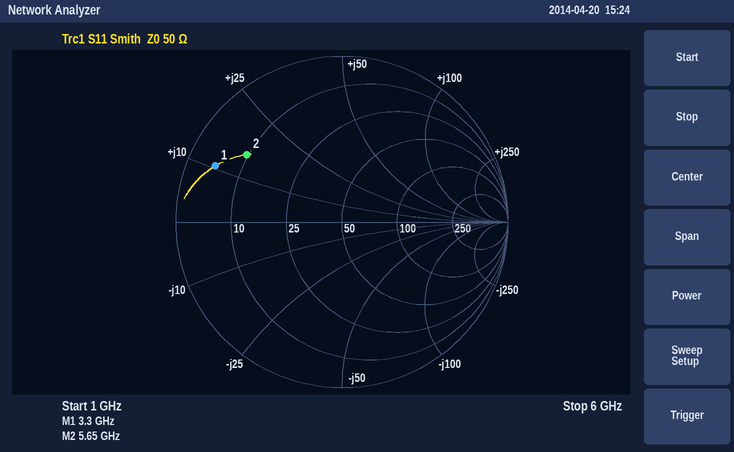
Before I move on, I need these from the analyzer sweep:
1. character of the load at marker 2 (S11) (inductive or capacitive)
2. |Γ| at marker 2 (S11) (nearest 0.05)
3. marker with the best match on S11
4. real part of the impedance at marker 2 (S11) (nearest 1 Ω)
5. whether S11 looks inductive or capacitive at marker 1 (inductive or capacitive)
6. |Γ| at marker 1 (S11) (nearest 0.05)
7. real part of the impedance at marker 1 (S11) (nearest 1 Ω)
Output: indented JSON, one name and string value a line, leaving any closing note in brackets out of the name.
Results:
{
  "character of the load at marker 2 (S11)": "inductive",
  "|Γ| at marker 2 (S11)": "0.70",
  "marker with the best match on S11": "marker 2",
  "real part of the impedance at marker 2 (S11)": "10 Ω",
  "whether S11 looks inductive or capacitive at marker 1": "inductive",
  "|Γ| at marker 1 (S11)": "0.85",
  "real part of the impedance at marker 1 (S11)": "5 Ω"
}
